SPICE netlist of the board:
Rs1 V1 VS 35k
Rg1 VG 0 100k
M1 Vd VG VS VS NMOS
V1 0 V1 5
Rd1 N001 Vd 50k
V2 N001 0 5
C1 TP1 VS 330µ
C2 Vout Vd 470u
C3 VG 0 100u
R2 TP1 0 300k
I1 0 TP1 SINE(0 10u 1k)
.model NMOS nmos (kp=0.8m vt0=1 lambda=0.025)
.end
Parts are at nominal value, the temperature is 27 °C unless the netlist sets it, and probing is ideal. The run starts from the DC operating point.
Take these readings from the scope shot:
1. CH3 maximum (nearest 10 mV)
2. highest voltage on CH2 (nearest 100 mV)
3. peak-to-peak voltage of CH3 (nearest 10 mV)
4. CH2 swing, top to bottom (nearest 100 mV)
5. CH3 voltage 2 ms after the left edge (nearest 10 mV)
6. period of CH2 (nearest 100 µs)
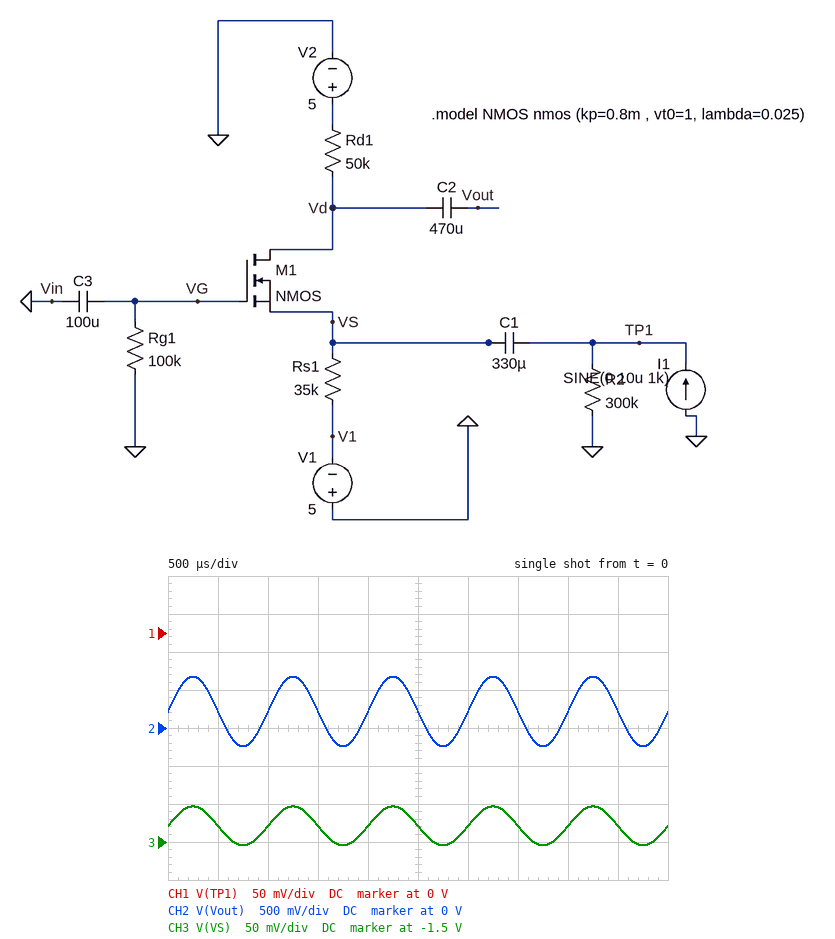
-1.45 V
700 mV
50 mV
900 mV
-1.48 V
1.0 ms
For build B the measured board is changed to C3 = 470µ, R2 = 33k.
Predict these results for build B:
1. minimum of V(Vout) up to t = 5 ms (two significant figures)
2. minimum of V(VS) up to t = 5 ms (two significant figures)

1.5 V
-1.4 V
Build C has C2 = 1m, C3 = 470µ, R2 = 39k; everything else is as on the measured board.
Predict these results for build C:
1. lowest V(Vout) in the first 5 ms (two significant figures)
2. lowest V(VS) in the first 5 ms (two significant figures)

1.2 V
-1.4 V
